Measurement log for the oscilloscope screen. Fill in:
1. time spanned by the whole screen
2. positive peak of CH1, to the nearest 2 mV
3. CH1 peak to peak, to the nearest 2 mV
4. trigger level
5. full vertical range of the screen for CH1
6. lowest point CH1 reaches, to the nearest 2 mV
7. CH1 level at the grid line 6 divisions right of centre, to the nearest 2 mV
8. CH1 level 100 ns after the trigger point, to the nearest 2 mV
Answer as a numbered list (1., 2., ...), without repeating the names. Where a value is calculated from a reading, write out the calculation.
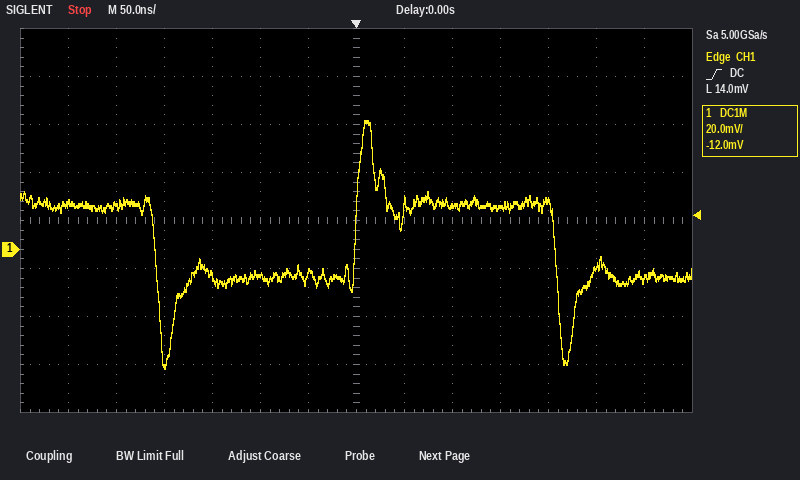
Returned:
1. 700 ns
2. 54 mV
3. 54 mV − (-50 mV) = 104 mV
4. 14.0 mV
5. 160 mV
6. -50 mV
7. -12 mV
8. 18 mV
